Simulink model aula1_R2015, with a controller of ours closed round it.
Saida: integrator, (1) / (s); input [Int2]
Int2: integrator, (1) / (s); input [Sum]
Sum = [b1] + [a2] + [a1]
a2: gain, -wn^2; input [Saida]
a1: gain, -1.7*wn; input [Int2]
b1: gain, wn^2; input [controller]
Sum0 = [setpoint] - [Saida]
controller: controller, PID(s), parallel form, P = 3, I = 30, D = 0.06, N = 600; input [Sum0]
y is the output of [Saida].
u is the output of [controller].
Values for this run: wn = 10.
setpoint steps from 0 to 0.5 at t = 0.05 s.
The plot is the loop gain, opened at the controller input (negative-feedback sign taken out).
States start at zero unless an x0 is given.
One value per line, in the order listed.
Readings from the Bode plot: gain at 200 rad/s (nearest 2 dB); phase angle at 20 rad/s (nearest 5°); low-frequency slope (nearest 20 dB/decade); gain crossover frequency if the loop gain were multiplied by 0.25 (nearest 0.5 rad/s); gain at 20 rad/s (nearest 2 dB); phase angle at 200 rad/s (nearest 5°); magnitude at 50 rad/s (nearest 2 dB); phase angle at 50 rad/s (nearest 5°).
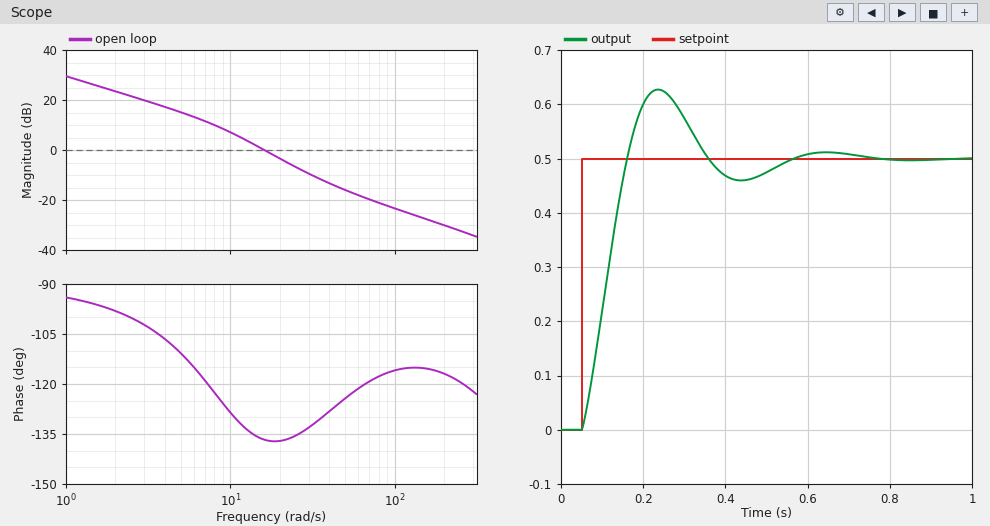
-30 dB
-135°
-20 dB/decade
6.5 rad/s
-4 dB
-115°
-16 dB
-125°
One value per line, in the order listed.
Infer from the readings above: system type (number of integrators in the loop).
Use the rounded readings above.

1
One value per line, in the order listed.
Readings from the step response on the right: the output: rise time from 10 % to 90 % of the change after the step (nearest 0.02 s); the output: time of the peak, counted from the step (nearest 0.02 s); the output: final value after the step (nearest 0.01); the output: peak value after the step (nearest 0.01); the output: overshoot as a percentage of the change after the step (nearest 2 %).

0.08 s
0.18 s
0.50
0.63
26 %
